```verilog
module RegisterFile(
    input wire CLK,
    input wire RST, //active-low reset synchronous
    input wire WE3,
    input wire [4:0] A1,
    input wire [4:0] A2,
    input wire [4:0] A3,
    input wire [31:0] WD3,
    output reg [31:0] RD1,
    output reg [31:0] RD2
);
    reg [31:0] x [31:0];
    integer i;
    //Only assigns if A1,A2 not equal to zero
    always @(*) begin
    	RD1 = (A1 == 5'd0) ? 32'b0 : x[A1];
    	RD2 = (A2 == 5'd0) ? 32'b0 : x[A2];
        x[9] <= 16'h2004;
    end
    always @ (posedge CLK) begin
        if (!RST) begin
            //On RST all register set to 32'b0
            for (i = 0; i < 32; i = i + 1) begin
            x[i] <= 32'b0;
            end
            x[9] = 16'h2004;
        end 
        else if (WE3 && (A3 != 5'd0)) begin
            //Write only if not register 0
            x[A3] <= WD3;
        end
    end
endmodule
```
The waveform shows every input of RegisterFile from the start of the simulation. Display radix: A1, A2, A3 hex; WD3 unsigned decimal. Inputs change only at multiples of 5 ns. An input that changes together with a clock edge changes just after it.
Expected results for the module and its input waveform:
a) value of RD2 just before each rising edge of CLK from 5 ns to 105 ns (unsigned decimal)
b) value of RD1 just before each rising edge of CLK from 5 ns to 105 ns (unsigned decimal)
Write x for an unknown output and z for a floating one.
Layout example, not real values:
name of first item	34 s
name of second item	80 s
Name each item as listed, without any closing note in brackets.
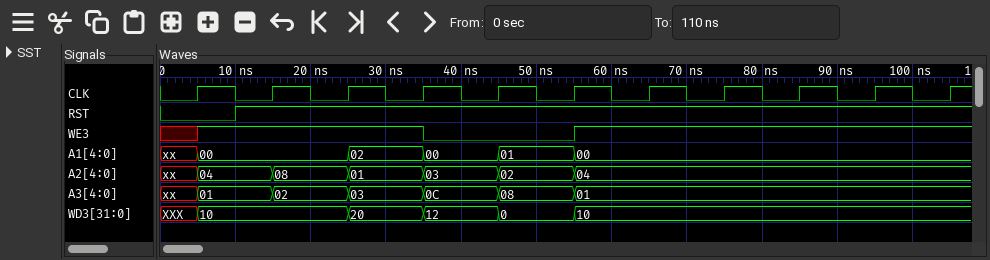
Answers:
value of RD2 just before each rising edge of CLK from 5 ns to 105 ns	x, 0, 0, 10, 20, 10, 0, 0, 0, 0, 0
value of RD1 just before each rising edge of CLK from 5 ns to 105 ns	x, 0, 0, 10, 0, 10, 0, 0, 0, 0, 0
